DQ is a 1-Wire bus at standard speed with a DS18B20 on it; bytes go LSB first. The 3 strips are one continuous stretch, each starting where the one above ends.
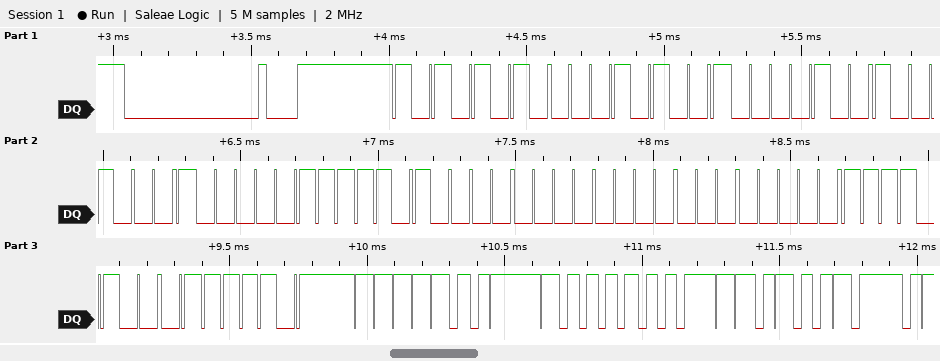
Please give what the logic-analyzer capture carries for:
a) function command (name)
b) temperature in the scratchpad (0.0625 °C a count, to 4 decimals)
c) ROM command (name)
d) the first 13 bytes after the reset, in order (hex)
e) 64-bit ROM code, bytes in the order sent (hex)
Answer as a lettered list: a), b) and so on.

a) Read Scratchpad
b) 25.9375 °C
c) Match ROM
d) 55 28 21 89 E0 0B 00 00 2F BE 9F 01 4B
e) 28 21 89 E0 0B 00 00 2F
